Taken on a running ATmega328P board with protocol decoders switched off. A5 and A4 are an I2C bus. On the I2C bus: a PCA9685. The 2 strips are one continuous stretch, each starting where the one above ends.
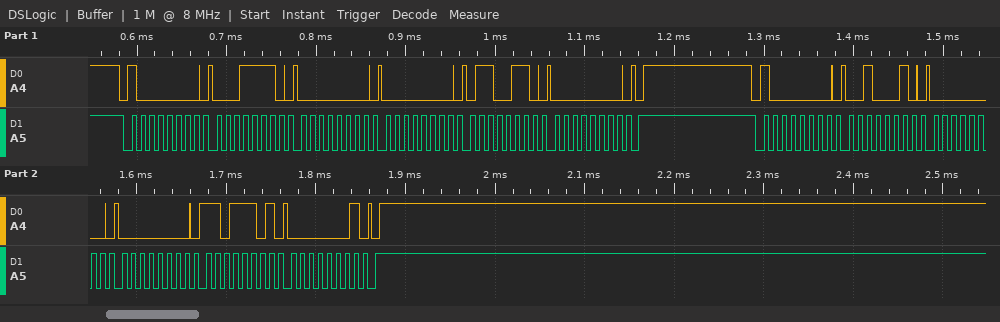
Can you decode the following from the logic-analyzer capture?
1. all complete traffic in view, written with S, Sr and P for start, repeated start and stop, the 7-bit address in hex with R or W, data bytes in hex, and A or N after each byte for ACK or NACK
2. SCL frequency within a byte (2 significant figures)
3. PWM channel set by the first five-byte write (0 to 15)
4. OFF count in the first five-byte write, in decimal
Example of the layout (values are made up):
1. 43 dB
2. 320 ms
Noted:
1. S 40W A 1E A 00 A 00 A 66 A 00 A P S 40W A 22 A 00 A 00 A DD A 01 A P
2. 100 kHz
3. 6
4. 102
